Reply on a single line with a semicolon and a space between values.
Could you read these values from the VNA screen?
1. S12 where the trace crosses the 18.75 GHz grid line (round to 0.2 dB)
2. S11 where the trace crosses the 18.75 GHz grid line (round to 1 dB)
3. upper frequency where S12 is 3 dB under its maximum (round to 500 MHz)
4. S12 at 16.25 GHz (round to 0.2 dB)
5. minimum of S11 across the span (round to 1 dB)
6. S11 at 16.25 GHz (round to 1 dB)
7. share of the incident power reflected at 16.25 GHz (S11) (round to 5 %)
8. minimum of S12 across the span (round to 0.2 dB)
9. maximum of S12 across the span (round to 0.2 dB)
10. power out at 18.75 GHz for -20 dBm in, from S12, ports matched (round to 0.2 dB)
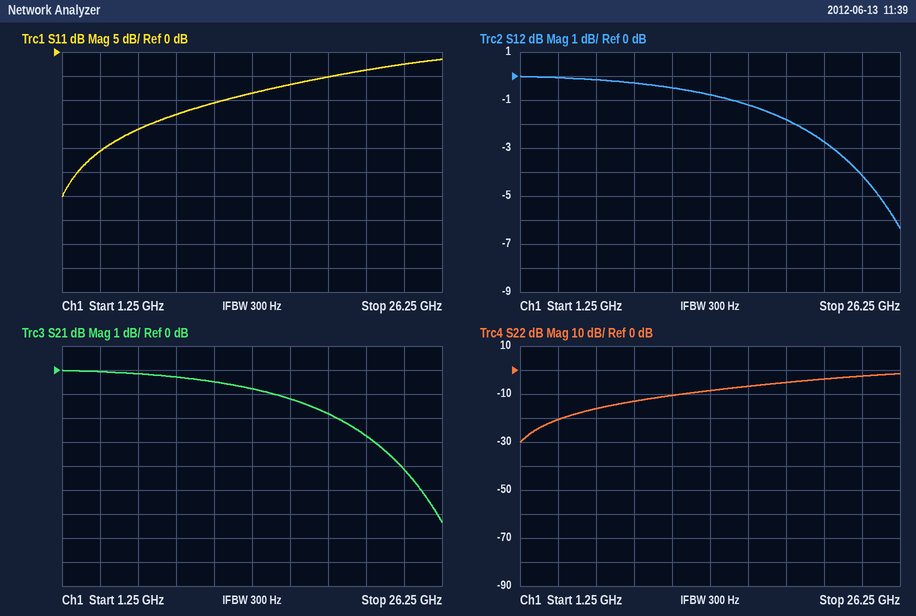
-1.8 dB; -5 dB; 22.0 GHz; -1.2 dB; -30 dB; -7 dB; 20 %; -6.4 dB; 0.0 dB; -21.8 dBm
